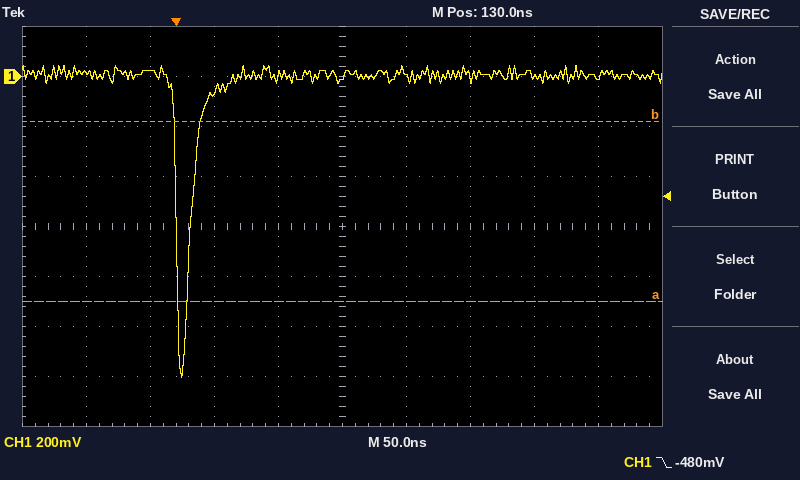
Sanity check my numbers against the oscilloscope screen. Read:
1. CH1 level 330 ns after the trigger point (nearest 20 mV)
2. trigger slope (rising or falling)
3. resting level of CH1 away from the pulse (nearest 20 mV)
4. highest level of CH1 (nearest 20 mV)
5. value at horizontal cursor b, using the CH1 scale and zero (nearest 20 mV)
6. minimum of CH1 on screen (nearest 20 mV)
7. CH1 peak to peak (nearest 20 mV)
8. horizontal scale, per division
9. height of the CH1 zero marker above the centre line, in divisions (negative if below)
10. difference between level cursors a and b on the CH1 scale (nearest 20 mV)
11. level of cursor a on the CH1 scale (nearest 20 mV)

0 mV
falling
0 mV
40 mV
-180 mV
-1.20 V
1.24 V
50 ns
+3.0 div
720 mV
-900 mV
